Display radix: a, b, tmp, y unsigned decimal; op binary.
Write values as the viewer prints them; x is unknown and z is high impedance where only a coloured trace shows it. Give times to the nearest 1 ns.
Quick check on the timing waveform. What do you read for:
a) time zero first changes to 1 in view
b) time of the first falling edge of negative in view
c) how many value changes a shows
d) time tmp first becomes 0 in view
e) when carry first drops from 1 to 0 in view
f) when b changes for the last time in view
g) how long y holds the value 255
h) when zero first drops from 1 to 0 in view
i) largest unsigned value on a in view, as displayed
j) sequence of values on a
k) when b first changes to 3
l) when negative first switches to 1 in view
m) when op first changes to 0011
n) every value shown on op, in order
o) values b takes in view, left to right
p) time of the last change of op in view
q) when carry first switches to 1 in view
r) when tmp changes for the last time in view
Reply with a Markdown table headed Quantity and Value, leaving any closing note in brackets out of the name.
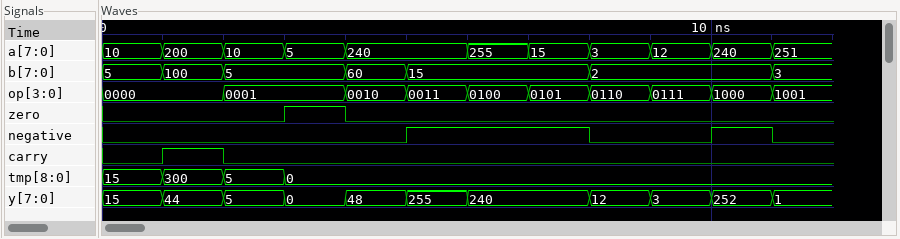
| Quantity | Value |
|---|---|
| time zero first changes to 1 in view | 3 ns |
| time of the first falling edge of negative in view | 8 ns |
| how many value changes a shows | 10 |
| time tmp first becomes 0 in view | 3 ns |
| when carry first drops from 1 to 0 in view | 2 ns |
| when b changes for the last time in view | 11 ns |
| how long y holds the value 255 | 1 ns |
| when zero first drops from 1 to 0 in view | 4 ns |
| largest unsigned value on a in view, as displayed | 255 |
| sequence of values on a | 10, 200, 10, 5, 240, 255, 15, 3, 12, 240, 251 |
| when b first changes to 3 | 11 ns |
| when negative first switches to 1 in view | 5 ns |
| when op first changes to 0011 | 5 ns |
| every value shown on op, in order | 0000, 0001, 0010, 0011, 0100, 0101, 0110, 0111, 1000, 1001 |
| values b takes in view, left to right | 5, 100, 5, 60, 15, 2, 3 |
| time of the last change of op in view | 11 ns |
| when carry first switches to 1 in view | 1 ns |
| when tmp changes for the last time in view | 3 ns |
